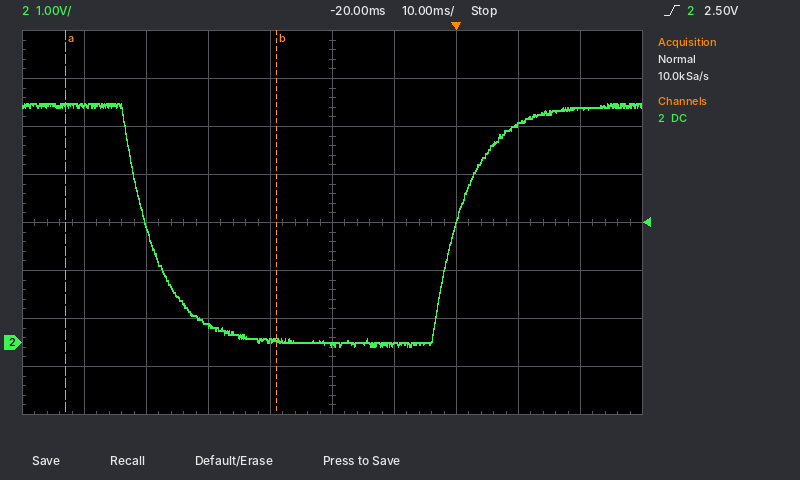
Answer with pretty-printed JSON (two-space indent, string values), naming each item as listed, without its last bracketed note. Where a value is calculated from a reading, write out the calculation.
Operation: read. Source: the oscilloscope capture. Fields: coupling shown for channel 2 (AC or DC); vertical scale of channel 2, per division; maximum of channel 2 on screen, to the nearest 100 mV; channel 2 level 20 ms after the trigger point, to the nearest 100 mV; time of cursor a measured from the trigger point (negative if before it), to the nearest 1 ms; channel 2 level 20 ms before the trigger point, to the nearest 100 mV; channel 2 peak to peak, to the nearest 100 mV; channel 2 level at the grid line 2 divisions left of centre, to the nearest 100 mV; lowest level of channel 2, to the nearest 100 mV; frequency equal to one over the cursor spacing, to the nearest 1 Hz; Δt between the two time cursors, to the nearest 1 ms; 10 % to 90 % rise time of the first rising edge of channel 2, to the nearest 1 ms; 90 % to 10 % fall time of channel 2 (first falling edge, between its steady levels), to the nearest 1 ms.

{
  "coupling shown for channel 2": "DC",
  "vertical scale of channel 2, per division": "1 V",
  "maximum of channel 2 on screen, to the nearest 100 mV": "5.0 V",
  "channel 2 level 20 ms after the trigger point, to the nearest 100 mV": "4.9 V",
  "time of cursor a measured from the trigger point (negative if before it), to the nearest 1 ms": "-63 ms",
  "channel 2 level 20 ms before the trigger point, to the nearest 100 mV": "0.0 V",
  "channel 2 peak to peak, to the nearest 100 mV": "5.0 V − (-100 mV) = 5.1 V",
  "channel 2 level at the grid line 2 divisions left of centre, to the nearest 100 mV": "400 mV",
  "lowest level of channel 2, to the nearest 100 mV": "-100 mV",
  "frequency equal to one over the cursor spacing, to the nearest 1 Hz": "1 / 34 ms ≈ 29 Hz",
  "Δt between the two time cursors, to the nearest 1 ms": "34 ms",
  "10 % to 90 % rise time of the first rising edge of channel 2, to the nearest 1 ms": "12 ms",
  "90 % to 10 % fall time of channel 2 (first falling edge, between its steady levels), to the nearest 1 ms": "12 ms"
}
